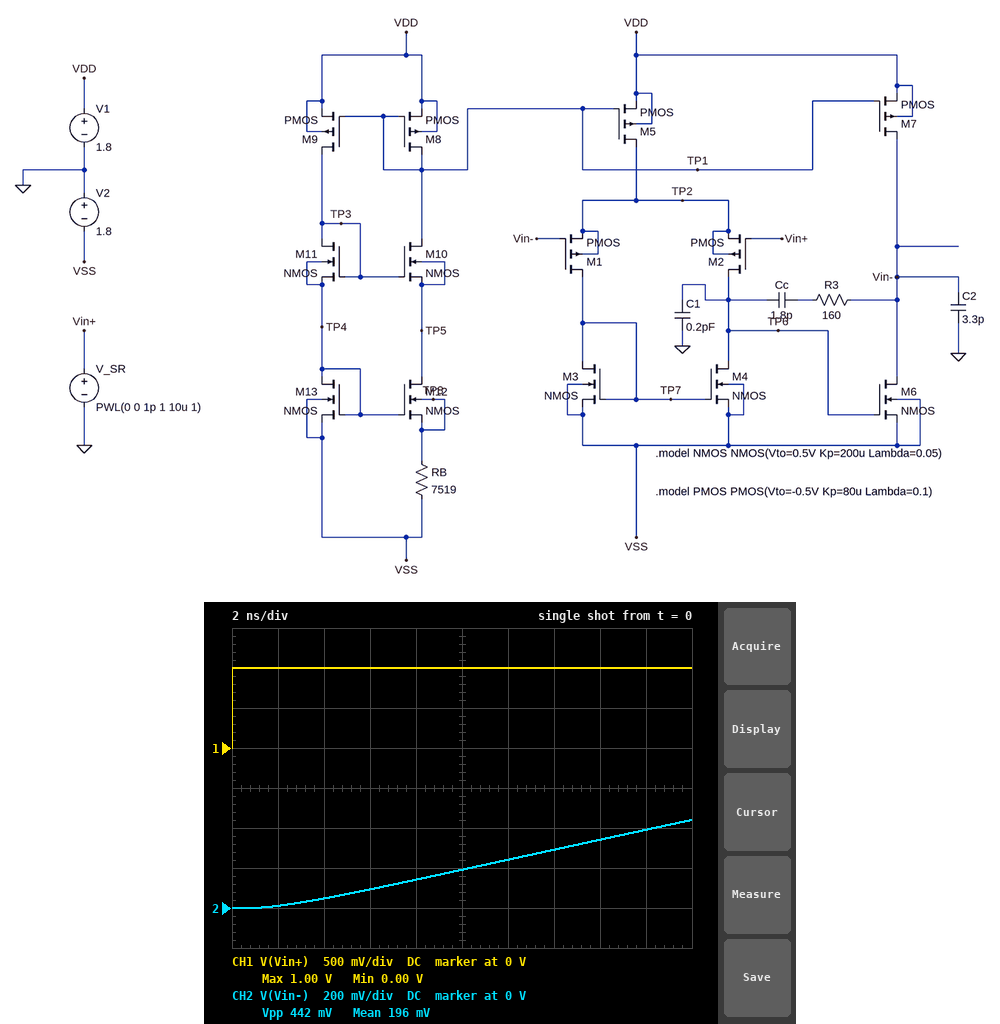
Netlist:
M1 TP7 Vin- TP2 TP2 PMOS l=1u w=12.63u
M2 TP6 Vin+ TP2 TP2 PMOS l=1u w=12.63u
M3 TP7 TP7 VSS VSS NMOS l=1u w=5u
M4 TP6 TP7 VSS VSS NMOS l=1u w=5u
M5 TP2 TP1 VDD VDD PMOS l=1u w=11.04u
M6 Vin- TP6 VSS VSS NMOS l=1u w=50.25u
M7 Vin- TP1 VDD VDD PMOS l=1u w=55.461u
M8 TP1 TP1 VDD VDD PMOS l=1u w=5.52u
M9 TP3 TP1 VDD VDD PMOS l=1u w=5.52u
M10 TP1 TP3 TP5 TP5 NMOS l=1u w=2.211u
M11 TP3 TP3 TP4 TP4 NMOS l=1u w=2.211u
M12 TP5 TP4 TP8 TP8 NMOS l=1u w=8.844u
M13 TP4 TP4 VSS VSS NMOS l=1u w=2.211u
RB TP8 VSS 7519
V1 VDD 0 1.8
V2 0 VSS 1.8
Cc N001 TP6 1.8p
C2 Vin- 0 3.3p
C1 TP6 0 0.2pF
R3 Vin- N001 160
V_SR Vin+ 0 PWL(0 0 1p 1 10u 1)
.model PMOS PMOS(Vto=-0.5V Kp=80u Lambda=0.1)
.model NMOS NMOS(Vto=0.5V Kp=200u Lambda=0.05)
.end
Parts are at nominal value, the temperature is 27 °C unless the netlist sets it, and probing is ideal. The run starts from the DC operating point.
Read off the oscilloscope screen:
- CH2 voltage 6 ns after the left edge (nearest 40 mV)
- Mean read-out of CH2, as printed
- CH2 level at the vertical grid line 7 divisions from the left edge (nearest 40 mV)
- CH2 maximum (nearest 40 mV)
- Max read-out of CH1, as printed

80 mV
196 mV
280 mV
440 mV
1.00 V
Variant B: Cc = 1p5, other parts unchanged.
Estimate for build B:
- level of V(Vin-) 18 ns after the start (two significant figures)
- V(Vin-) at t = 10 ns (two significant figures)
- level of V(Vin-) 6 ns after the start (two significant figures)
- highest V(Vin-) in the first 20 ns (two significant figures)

470 mV
230 mV
110 mV
530 mV
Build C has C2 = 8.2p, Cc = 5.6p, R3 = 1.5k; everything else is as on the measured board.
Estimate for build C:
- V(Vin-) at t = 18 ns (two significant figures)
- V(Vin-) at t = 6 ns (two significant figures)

160 mV
57 mV
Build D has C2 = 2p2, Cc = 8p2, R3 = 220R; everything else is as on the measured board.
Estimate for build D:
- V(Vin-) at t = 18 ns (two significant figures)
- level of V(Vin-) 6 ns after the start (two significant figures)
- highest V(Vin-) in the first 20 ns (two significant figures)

84 mV
17 mV
96 mV
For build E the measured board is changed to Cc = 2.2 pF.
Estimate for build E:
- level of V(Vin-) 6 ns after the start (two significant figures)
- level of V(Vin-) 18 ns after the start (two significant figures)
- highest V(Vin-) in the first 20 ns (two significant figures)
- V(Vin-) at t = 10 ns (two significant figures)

75 mV
320 mV
360 mV
160 mV
